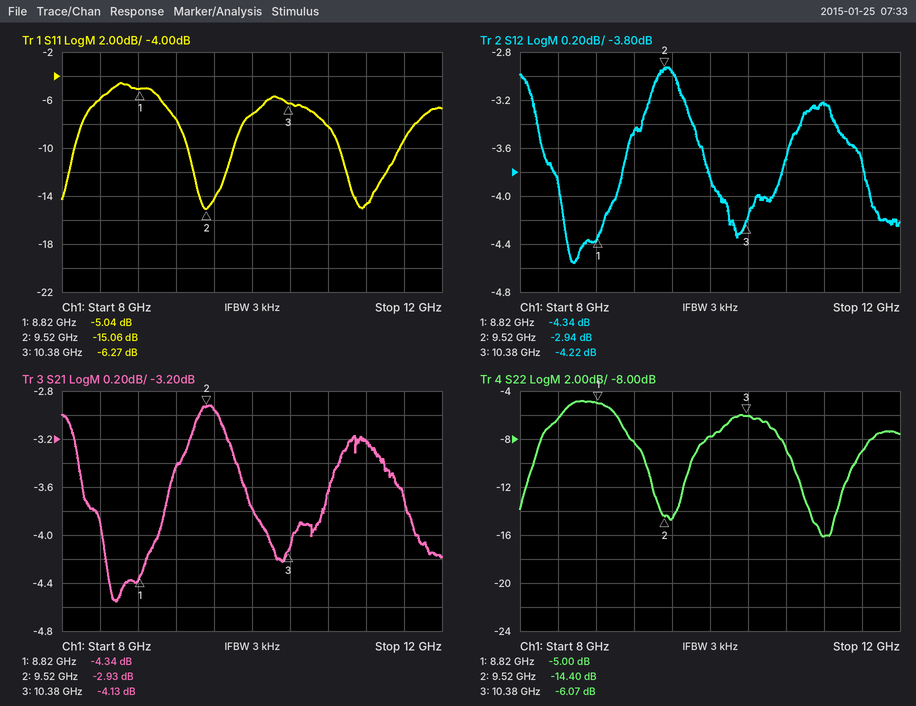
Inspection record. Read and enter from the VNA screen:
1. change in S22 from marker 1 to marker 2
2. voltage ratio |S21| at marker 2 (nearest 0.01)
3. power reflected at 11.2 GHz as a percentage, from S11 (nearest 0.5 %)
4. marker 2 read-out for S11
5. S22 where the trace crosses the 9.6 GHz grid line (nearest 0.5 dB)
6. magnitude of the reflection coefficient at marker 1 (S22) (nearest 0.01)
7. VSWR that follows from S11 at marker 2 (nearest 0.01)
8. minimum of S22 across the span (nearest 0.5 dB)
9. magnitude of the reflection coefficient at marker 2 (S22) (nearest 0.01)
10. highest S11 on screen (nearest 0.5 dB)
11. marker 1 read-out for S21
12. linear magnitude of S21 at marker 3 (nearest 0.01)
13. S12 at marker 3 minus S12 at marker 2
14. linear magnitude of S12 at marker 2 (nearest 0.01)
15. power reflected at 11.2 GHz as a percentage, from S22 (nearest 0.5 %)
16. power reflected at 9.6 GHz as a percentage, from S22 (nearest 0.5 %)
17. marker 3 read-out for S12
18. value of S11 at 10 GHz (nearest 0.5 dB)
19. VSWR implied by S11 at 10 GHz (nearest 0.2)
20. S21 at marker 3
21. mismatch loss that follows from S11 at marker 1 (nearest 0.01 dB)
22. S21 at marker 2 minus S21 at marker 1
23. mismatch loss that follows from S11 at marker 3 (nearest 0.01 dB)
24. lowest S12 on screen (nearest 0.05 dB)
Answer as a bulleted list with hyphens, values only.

- -9.40 dB
- 0.71
- 3.5 %
- -15.06 dB
- -14.5 dB
- 0.56
- 1.43
- -16.0 dB
- 0.19
- -4.5 dB
- -4.34 dB
- 0.62
- -1.28 dB
- 0.71
- 2.5 %
- 3.5 %
- -4.22 dB
- -7.0 dB
- 2.6
- -4.13 dB
- 1.63 dB
- 1.41 dB
- 1.17 dB
- -4.55 dB
